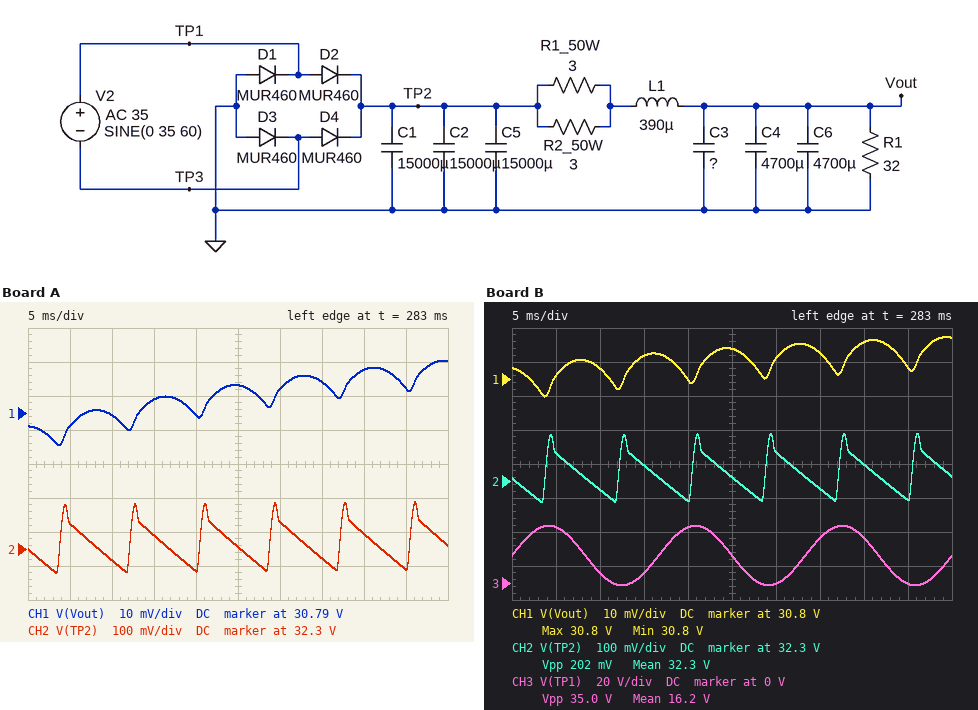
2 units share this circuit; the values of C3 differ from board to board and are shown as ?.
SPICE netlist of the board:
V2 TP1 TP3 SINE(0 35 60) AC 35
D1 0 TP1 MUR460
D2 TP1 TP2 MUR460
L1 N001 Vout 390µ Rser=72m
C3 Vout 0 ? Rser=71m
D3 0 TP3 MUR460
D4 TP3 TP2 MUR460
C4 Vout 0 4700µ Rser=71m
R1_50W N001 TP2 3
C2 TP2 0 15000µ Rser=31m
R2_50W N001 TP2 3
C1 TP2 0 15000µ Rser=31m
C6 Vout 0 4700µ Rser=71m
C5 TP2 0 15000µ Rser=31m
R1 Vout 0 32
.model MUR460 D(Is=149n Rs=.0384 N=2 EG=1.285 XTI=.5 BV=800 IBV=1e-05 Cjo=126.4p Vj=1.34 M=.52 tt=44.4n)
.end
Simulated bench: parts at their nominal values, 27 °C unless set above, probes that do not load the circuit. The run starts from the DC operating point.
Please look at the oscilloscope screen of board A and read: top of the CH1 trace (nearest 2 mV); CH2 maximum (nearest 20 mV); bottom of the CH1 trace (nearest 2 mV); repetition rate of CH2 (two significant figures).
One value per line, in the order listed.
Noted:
30.806 V
32.44 V
30.780 V
120 Hz
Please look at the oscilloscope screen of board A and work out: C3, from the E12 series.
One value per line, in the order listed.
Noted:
5.6 mF
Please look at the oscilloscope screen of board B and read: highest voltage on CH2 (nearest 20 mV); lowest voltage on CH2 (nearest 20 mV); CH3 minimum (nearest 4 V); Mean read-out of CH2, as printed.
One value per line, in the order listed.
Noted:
32.44 V
32.24 V
0 V
32.3 V
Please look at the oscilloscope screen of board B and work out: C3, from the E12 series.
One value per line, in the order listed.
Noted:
2.7 mF
